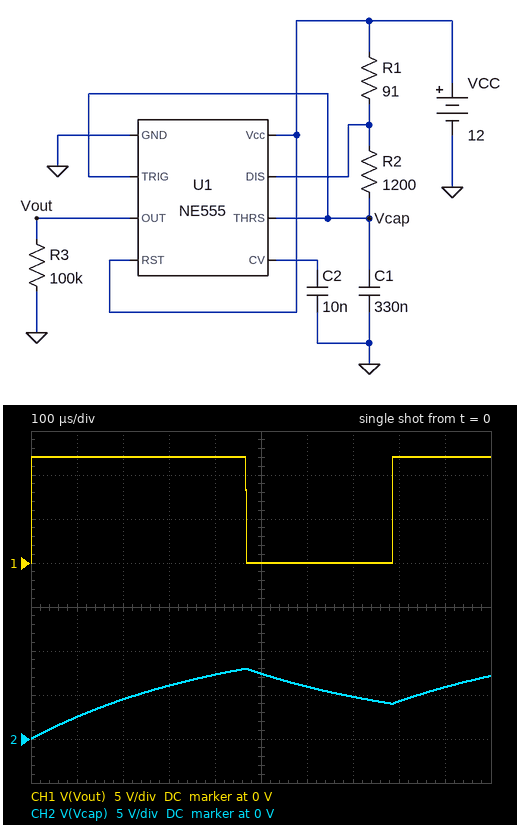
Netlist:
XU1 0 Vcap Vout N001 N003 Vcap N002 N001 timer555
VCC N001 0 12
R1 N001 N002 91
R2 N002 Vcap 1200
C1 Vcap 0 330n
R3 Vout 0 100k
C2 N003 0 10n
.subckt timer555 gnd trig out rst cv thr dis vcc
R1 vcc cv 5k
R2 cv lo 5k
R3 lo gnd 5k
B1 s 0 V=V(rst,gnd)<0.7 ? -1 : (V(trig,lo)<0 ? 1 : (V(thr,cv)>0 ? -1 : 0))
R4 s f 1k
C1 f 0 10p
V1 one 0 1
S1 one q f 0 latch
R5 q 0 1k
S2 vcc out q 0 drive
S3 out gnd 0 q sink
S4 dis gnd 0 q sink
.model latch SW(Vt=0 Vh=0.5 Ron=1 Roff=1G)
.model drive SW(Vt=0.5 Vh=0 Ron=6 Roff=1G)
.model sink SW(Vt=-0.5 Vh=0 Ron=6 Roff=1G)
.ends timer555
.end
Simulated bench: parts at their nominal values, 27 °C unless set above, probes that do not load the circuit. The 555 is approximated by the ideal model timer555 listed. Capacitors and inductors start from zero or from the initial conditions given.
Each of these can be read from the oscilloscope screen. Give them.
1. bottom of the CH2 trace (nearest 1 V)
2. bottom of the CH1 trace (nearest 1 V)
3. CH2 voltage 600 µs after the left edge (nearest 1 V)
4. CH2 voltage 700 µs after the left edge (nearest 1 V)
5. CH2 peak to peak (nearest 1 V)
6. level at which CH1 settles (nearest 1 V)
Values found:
0 V
0 V
6 V
5 V
8 V
12 V
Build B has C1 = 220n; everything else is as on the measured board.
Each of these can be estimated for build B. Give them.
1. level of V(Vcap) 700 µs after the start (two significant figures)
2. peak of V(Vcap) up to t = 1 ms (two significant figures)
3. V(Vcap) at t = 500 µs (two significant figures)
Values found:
7.7 V
8.0 V
4.3 V
